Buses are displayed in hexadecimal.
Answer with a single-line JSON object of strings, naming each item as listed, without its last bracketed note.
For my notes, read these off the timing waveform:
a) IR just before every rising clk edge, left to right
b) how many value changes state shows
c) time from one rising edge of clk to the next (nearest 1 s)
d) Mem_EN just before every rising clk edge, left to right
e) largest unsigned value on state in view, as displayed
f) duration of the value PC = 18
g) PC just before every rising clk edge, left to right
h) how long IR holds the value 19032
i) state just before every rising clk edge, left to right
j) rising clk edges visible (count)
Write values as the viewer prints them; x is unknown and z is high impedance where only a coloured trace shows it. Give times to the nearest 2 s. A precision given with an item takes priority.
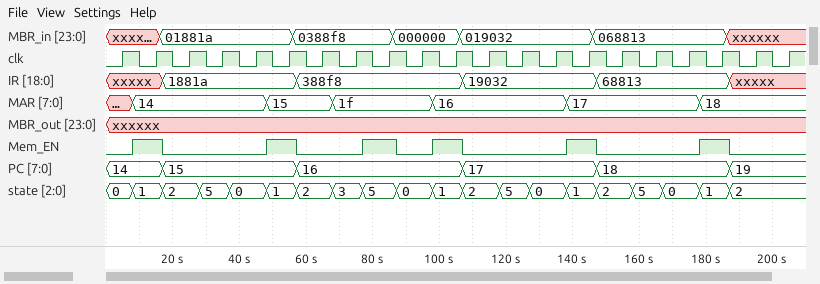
{"IR just before every rising clk edge, left to right": "xxxxx, xxxxx, 1881a, 1881a, 1881a, 1881a, 388f8, 388f8, 388f8, 388f8, 388f8, 19032, 19032, 19032, 19032, 68813, 68813, 68813, 68813, xxxxx, xxxxx", "how many value changes state shows": "19", "time from one rising edge of clk to the next": "10 s", "Mem_EN just before every rising clk edge, left to right": "0 1 0 0 0 1 0 0 1 0 1 0 0 0 1 0 0 0 1 0 0", "largest unsigned value on state in view, as displayed": "5", "duration of the value PC = 18": "40 s", "PC just before every rising clk edge, left to right": "14, 14, 15, 15, 15, 15, 16, 16, 16, 16, 16, 17, 17, 17, 17, 18, 18, 18, 18, 19, 19", "how long IR holds the value 19032": "40 s", "state just before every rising clk edge, left to right": "0, 1, 2, 5, 0, 1, 2, 3, 5, 0, 1, 2, 5, 0, 1, 2, 5, 0, 1, 2, 2", "rising clk edges visible": "21"}
